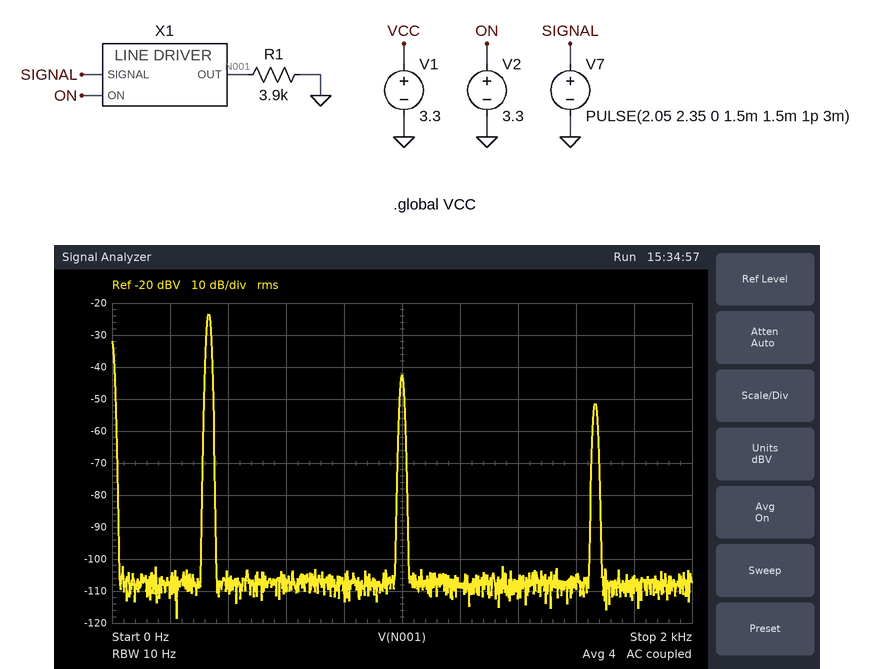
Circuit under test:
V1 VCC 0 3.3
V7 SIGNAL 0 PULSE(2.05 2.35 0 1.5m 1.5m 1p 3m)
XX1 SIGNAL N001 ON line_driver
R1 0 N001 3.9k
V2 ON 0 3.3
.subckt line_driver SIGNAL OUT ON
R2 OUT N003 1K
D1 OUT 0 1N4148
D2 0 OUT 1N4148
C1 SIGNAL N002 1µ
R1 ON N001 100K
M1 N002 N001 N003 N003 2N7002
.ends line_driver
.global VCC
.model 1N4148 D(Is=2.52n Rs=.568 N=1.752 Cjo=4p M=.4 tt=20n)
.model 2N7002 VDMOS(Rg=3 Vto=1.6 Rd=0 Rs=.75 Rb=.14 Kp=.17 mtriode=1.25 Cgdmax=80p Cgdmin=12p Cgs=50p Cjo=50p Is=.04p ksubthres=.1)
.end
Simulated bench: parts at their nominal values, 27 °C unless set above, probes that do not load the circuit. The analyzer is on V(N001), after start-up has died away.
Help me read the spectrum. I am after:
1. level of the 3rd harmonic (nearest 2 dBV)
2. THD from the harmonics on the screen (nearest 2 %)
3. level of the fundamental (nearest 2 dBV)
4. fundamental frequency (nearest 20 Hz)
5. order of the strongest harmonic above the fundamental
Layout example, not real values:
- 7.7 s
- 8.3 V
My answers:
- -42 dBV
- 12 %
- -24 dBV
- 340 Hz
- 3
